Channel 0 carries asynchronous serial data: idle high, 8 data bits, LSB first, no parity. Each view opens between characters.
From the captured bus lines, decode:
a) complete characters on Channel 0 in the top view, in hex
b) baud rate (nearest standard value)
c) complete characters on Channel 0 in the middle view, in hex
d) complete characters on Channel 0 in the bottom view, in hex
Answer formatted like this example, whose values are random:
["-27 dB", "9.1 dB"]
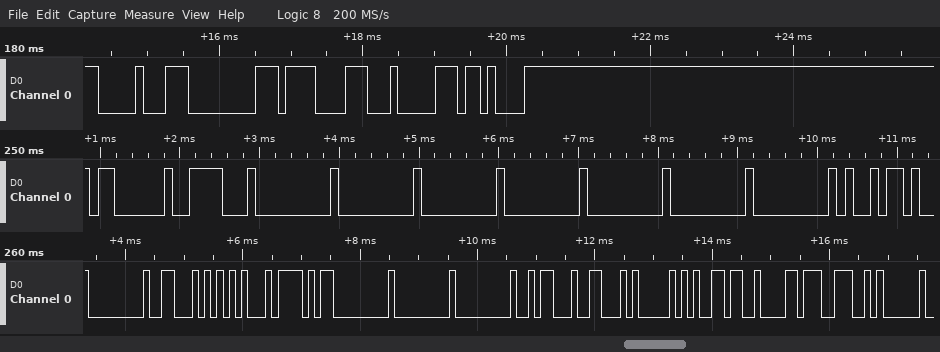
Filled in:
["10, 00, 0F, 04, 0B", "9600 baud", "03, 1E, 00, 00, 00, 00, 00, 00, 00, 69", "00, 46, 15, AF, 00, 00, 00, 1A, 46, 50, 36, D8, 4E"]
